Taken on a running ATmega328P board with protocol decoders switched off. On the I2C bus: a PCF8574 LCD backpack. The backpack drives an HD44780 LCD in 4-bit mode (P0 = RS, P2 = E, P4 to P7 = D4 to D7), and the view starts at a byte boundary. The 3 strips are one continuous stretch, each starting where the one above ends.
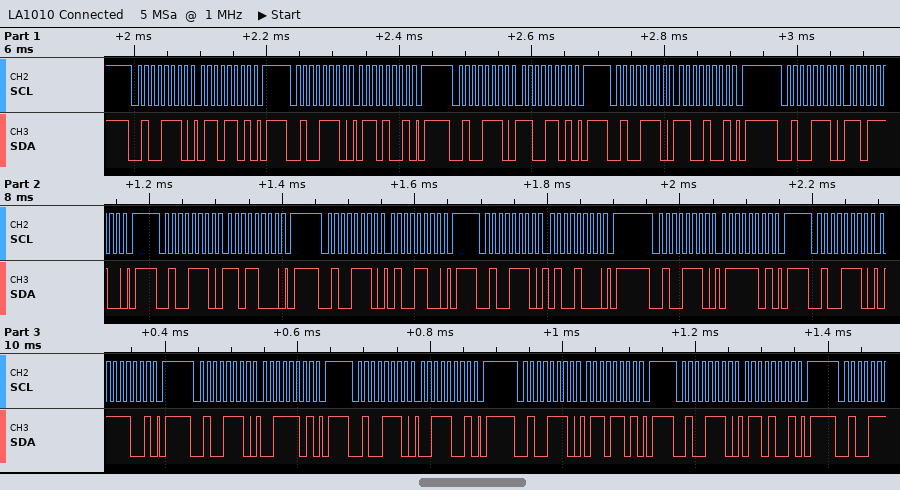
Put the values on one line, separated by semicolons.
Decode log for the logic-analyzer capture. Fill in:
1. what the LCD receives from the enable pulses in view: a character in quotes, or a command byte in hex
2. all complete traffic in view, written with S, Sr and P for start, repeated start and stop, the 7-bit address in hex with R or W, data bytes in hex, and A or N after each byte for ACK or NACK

'l' 0xD4 's'; S 27W A 6D A P S 27W A 69 A P S 27W A CD A P S 27W A C9 A P S 27W A DC A P S 27W A D8 A P S 27W A 4C A P S 27W A 48 A P S 27W A 7D A P S 27W A 79 A P S 27W A 3D A P S 27W A 39 A P S 27W A 6D A P S 27W A 69 A P
